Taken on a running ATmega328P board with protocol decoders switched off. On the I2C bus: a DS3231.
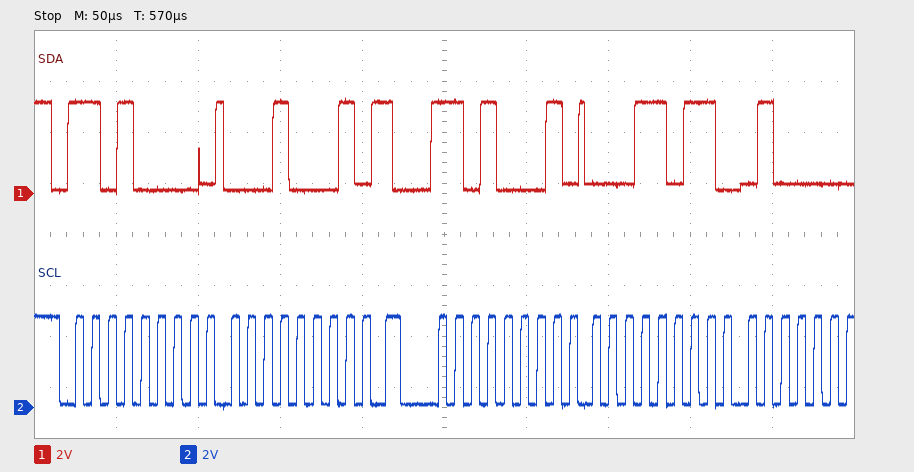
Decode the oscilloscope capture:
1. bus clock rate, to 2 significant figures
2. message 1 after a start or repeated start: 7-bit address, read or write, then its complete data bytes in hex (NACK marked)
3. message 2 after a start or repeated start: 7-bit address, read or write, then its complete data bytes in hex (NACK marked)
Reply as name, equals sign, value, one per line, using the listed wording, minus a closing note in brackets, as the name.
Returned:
bus clock rate, to 2 significant figures = 100 kHz
message 1 after a start or repeated start: 7-bit address, read or write, then its complete data bytes in hex = 0x68 write: 11
message 2 after a start or repeated start: 7-bit address, read or write, then its complete data bytes in hex = 0x68 read: 1B
